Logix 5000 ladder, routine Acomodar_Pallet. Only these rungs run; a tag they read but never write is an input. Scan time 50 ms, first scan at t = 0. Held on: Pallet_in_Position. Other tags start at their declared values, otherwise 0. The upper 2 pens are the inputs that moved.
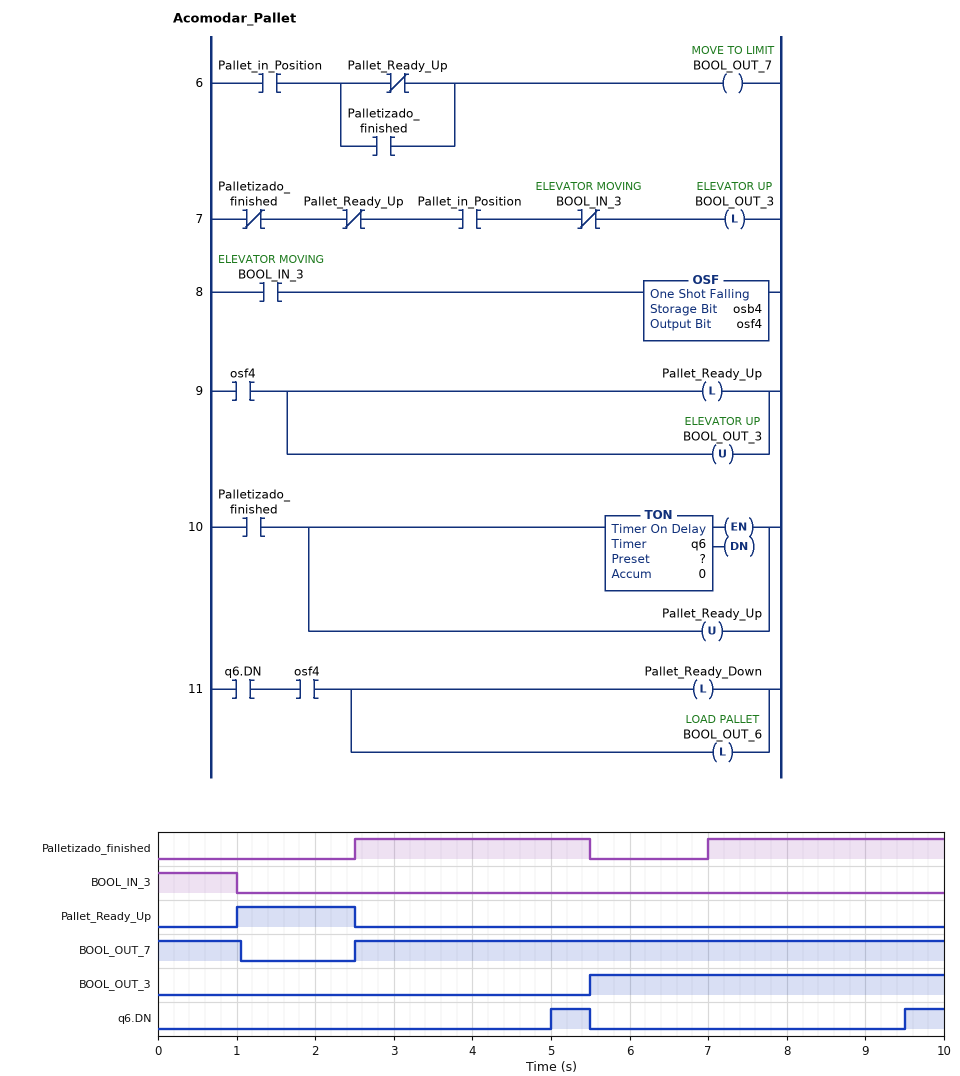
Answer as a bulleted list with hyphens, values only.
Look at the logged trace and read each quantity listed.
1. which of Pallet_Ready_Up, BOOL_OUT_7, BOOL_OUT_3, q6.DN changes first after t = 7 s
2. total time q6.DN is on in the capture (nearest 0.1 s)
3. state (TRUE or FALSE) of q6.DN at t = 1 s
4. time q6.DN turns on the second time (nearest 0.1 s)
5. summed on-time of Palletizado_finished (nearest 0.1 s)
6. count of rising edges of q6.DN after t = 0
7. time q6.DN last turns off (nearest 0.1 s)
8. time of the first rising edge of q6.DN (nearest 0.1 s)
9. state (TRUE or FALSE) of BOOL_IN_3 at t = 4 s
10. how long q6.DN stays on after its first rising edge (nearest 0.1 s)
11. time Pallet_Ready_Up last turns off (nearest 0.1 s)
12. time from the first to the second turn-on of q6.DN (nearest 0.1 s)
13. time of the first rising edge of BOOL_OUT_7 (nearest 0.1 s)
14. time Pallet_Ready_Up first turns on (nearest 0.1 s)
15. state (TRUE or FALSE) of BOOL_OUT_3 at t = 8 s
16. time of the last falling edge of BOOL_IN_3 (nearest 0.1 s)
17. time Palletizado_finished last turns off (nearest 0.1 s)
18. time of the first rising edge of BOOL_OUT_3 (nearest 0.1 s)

- q6.DN
- 1.0 s
- FALSE
- 9.5 s
- 6.0 s
- 2
- 5.5 s
- 5.0 s
- FALSE
- 0.5 s
- 2.5 s
- 4.5 s
- 2.5 s
- 1.0 s
- TRUE
- 1.0 s
- 5.5 s
- 5.5 s
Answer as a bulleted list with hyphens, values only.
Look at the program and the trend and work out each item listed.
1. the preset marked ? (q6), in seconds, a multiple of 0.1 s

- 2.5 s
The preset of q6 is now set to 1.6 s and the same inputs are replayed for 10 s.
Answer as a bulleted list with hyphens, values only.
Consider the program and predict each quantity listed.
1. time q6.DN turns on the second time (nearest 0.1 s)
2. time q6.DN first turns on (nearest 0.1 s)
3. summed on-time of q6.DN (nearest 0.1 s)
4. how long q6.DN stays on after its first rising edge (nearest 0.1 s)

- 8.6 s
- 4.1 s
- 2.8 s
- 1.4 s
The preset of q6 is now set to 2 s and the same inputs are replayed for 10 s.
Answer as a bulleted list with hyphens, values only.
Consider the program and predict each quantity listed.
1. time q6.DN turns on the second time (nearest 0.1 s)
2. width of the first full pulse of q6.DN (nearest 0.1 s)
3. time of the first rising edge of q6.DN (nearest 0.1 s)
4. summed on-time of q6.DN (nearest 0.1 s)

- 9.0 s
- 1.0 s
- 4.5 s
- 2.0 s
